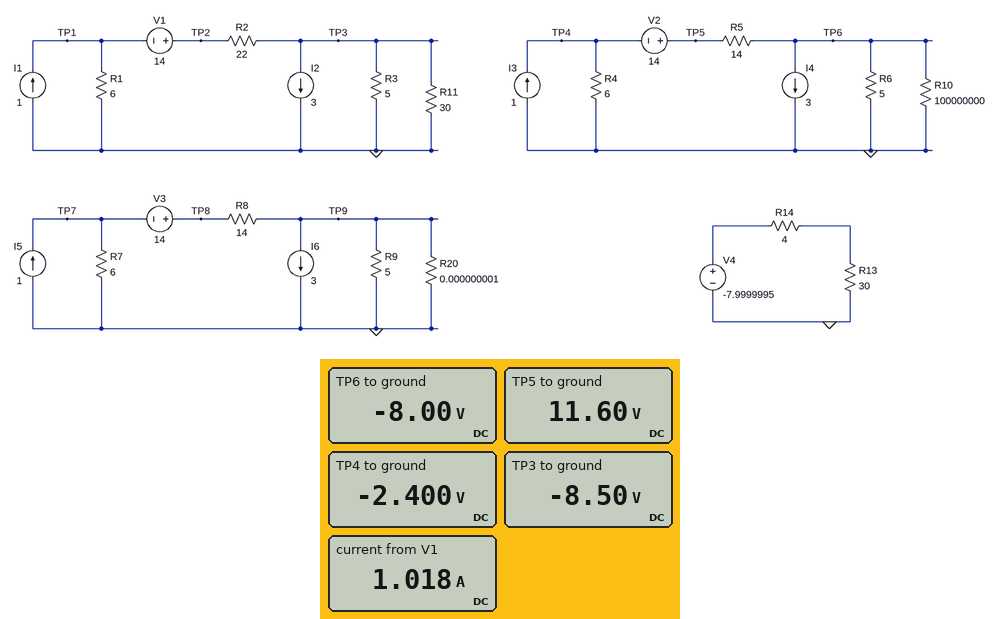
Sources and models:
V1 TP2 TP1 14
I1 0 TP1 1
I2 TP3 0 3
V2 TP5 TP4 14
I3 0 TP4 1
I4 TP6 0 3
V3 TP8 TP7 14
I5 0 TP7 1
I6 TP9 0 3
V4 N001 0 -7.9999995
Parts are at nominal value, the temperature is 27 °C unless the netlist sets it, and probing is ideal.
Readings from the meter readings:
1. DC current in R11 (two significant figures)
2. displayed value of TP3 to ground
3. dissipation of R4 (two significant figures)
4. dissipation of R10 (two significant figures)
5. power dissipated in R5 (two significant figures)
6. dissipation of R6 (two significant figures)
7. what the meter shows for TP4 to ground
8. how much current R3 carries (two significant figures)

280 mA
-8.50 V
960 mW
640 nW
27 W
13 W
-2.400 V
1.7 A
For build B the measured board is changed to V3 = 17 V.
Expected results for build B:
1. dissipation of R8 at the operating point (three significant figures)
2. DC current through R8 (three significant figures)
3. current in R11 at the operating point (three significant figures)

18.5 W
1.15 A
283 mA
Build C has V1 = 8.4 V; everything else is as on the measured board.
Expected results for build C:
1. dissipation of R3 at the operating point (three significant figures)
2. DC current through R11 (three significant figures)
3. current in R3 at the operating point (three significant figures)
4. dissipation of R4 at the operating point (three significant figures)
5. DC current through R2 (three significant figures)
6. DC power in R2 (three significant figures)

17.1 W
308 mA
1.85 A
960 mW
844 mA
15.7 W
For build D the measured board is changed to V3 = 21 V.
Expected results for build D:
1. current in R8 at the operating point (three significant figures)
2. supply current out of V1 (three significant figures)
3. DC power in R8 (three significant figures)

1.35 A
1.02 A
25.5 W
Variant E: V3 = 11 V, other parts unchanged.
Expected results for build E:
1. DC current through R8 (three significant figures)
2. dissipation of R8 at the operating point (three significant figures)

850 mA
10.1 W
